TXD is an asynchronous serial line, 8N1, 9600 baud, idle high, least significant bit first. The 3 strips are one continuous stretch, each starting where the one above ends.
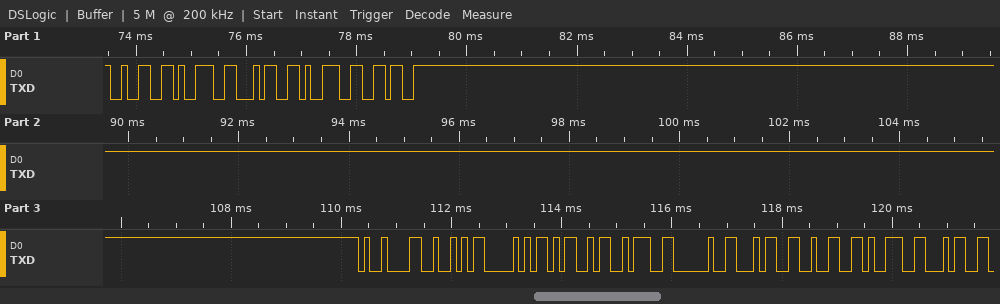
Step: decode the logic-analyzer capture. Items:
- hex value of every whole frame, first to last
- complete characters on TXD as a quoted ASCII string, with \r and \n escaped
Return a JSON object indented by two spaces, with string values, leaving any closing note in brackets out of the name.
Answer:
{
  "hex value of every whole frame, first to last": "32 39 34 39 36 09 52 50 4D 3A 20 34 32 39 34",
  "complete characters on TXD as a quoted ASCII string, with \\r and \\n escaped": "\"29496\\tRPM: 4294\""
}
